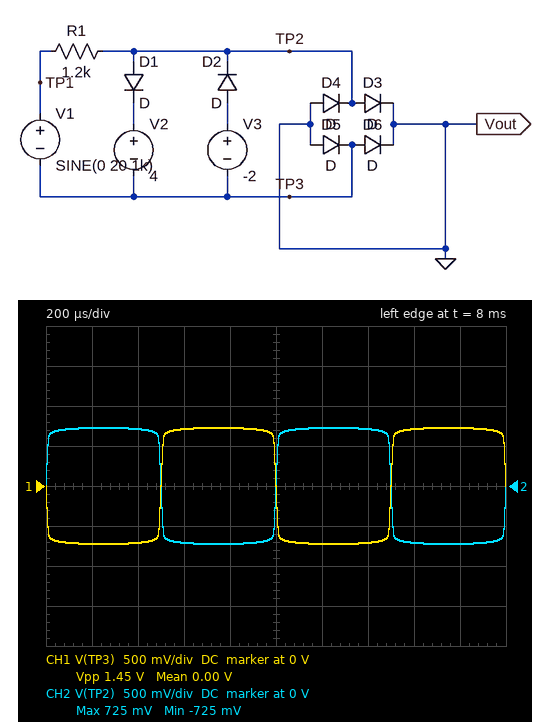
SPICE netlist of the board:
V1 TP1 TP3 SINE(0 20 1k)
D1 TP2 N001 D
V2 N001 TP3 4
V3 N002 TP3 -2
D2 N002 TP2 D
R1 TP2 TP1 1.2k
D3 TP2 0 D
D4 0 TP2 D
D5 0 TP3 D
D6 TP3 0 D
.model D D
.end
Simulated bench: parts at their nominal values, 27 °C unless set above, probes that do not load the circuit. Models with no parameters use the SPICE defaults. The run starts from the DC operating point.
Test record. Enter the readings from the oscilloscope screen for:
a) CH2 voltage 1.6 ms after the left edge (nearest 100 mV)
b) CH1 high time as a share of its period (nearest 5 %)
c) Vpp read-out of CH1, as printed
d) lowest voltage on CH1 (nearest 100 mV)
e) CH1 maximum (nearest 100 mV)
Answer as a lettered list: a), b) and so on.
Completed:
a) -700 mV
b) 50 %
c) 1.45 V
d) -700 mV
e) 700 mV
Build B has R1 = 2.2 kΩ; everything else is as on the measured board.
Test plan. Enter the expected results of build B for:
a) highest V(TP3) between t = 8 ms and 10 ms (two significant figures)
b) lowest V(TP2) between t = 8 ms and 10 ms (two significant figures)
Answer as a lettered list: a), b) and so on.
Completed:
a) 710 mV
b) -710 mV
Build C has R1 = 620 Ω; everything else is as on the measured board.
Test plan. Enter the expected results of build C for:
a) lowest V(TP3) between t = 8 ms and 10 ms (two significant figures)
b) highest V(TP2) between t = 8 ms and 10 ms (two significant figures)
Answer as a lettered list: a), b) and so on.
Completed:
a) -740 mV
b) 740 mV
